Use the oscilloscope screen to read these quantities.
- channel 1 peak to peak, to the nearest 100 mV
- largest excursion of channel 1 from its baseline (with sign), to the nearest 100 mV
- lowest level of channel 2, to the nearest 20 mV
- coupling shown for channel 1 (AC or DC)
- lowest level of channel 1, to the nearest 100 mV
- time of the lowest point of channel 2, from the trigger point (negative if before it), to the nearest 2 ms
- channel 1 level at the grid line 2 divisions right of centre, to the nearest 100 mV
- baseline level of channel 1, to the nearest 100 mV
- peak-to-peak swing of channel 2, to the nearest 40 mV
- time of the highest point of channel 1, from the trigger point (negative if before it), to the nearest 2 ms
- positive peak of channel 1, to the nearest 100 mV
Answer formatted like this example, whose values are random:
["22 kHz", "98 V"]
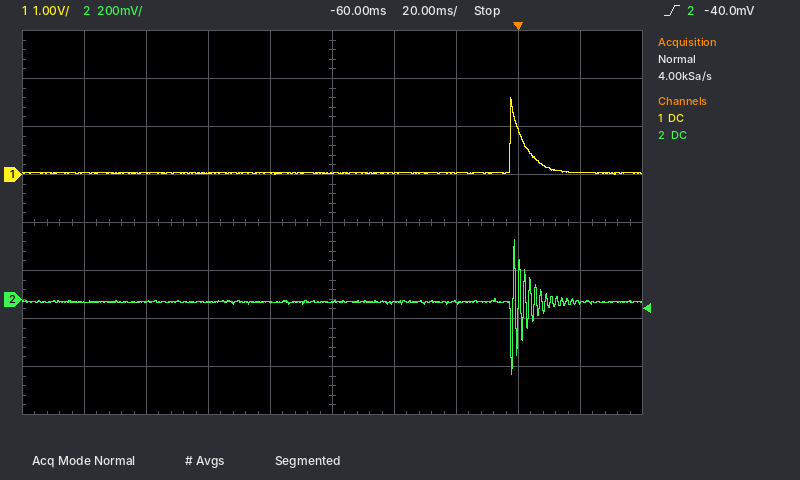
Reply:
["1.6 V", "+1.6 V", "-320 mV", "DC", "0.0 V", "-2 ms", "0.0 V", "0.0 V", "560 mV", "-2 ms", "1.6 V"]
